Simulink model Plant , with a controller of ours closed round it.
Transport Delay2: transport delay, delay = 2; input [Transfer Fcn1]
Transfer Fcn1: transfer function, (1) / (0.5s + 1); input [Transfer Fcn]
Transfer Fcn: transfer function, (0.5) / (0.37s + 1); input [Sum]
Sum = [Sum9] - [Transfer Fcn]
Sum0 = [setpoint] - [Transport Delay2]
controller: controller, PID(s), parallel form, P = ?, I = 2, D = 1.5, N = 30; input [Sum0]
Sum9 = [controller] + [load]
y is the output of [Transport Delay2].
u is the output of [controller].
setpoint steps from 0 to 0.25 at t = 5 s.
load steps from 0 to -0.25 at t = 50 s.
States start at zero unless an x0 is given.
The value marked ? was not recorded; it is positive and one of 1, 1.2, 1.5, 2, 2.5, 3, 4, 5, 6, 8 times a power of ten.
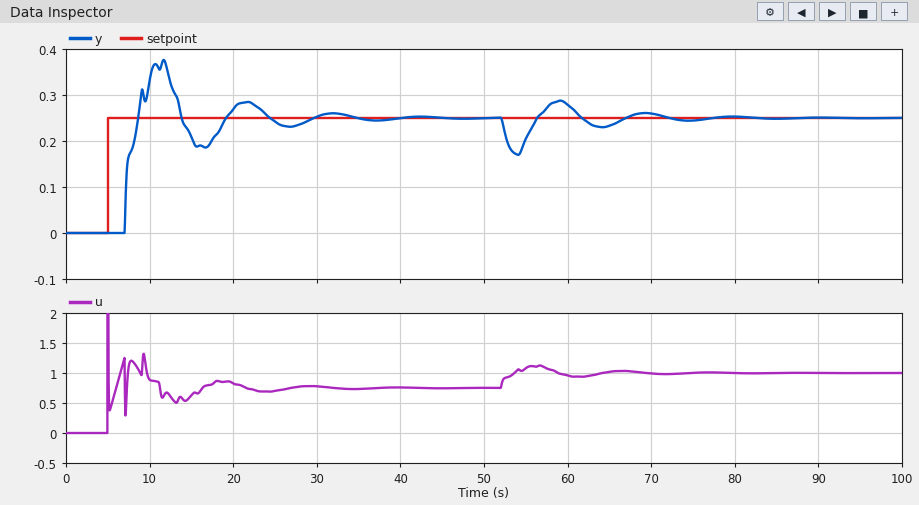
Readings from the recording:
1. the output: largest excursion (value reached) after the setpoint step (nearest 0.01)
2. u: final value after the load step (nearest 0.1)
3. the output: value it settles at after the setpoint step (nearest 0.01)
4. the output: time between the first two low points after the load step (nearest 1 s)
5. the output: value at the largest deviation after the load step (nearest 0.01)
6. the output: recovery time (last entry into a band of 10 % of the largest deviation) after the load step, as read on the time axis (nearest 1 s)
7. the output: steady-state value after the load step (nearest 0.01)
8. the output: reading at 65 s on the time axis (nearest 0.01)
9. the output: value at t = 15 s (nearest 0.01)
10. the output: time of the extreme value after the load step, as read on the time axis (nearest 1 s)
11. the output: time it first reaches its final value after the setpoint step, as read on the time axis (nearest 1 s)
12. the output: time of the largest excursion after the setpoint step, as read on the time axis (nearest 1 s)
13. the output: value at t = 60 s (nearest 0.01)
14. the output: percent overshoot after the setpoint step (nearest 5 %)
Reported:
0.38
1.0
0.25
10 s
0.17
71 s
0.25
0.23
0.21
54 s
9 s
12 s
0.28
50 %
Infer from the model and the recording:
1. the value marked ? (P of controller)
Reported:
1
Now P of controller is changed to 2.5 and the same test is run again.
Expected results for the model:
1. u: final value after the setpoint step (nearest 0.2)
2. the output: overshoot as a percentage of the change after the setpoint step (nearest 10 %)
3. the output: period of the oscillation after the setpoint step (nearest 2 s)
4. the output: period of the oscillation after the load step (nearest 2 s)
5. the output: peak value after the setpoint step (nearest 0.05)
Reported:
0.8
70 %
6 s
6 s
0.45
